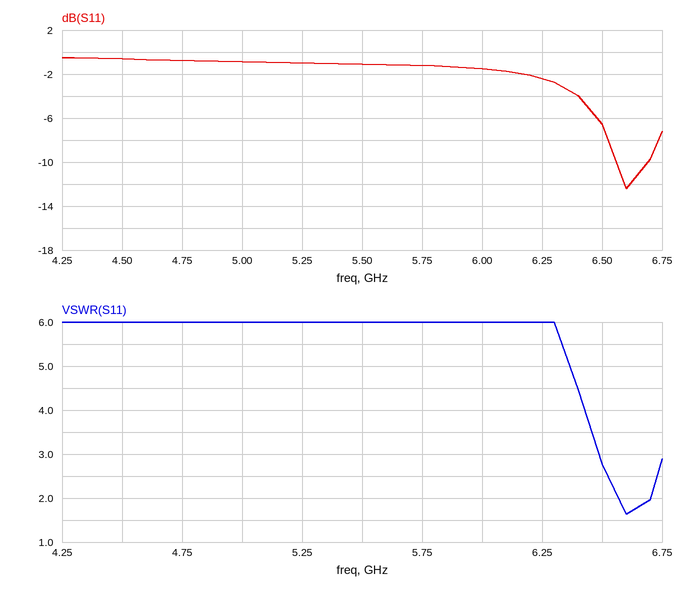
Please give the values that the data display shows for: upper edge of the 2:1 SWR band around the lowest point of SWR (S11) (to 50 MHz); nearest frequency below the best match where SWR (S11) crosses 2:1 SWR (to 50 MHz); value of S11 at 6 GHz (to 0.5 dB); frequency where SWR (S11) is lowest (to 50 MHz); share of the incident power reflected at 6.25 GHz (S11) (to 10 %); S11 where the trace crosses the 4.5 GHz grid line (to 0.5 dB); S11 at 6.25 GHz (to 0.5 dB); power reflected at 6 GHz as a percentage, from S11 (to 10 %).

6.70 GHz
6.55 GHz
-1.5 dB
6.60 GHz
60 %
-0.5 dB
-2.5 dB
70 %
